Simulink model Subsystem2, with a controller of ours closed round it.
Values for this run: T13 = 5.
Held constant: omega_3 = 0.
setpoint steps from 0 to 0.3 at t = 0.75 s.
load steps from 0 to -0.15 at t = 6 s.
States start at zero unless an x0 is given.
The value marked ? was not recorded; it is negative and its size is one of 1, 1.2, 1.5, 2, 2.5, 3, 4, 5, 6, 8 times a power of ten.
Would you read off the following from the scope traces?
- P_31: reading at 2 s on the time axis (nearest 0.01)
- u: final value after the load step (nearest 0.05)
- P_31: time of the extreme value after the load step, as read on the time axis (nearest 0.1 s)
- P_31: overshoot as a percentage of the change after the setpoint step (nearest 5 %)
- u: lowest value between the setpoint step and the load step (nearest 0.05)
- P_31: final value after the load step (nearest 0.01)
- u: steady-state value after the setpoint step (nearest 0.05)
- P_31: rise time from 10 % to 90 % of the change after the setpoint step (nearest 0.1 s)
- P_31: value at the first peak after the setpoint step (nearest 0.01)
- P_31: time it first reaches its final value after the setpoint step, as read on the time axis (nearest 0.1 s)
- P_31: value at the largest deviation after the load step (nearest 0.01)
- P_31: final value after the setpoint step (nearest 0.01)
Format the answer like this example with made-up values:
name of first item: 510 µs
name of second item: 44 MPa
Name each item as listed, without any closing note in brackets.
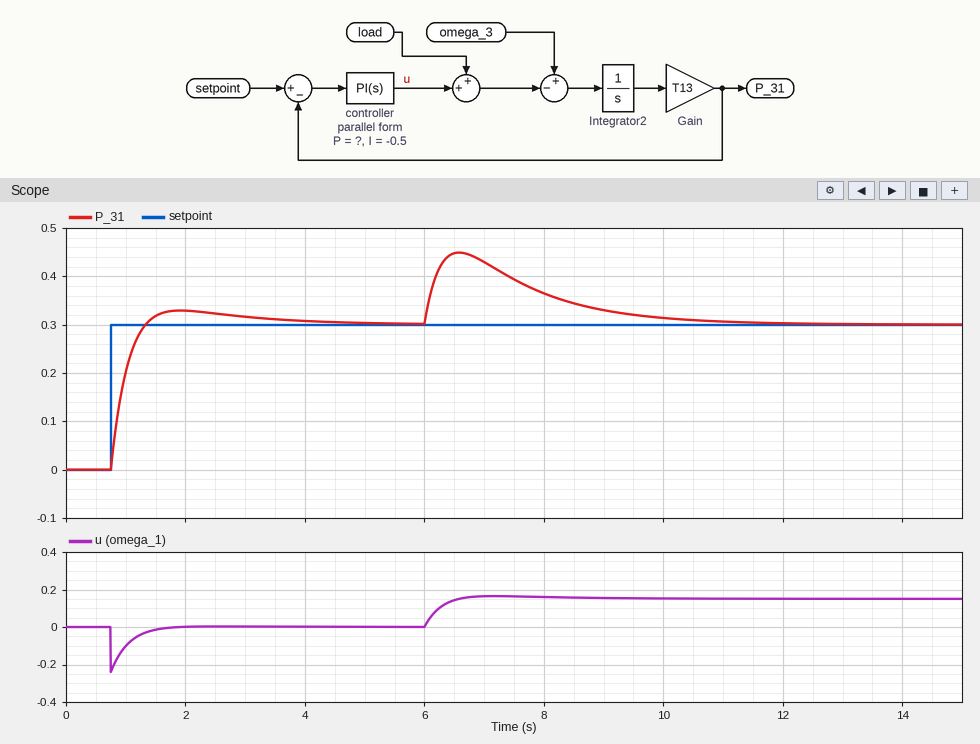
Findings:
P_31: reading at 2 s on the time axis: 0.33
u: final value after the load step: 0.15
P_31: time of the extreme value after the load step, as read on the time axis: 6.6 s
P_31: overshoot as a percentage of the change after the setpoint step: 10 %
u: lowest value between the setpoint step and the load step: -0.25
P_31: final value after the load step: 0.30
u: steady-state value after the setpoint step: 0.00
P_31: rise time from 10 % to 90 % of the change after the setpoint step: 0.4 s
P_31: value at the first peak after the setpoint step: 0.33
P_31: time it first reaches its final value after the setpoint step, as read on the time axis: 1.3 s
P_31: value at the largest deviation after the load step: 0.45
P_31: final value after the setpoint step: 0.30
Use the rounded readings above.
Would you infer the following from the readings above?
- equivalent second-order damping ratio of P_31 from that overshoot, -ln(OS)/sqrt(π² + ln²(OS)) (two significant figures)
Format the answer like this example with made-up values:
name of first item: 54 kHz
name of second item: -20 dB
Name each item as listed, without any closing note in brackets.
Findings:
equivalent second-order damping ratio of P_31 from that overshoot, -ln(OS)/sqrt(π² + ln²(OS)): 0.59
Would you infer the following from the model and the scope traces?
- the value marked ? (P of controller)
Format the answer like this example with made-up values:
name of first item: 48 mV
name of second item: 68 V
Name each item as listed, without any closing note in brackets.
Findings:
the value marked ?: -0.8
